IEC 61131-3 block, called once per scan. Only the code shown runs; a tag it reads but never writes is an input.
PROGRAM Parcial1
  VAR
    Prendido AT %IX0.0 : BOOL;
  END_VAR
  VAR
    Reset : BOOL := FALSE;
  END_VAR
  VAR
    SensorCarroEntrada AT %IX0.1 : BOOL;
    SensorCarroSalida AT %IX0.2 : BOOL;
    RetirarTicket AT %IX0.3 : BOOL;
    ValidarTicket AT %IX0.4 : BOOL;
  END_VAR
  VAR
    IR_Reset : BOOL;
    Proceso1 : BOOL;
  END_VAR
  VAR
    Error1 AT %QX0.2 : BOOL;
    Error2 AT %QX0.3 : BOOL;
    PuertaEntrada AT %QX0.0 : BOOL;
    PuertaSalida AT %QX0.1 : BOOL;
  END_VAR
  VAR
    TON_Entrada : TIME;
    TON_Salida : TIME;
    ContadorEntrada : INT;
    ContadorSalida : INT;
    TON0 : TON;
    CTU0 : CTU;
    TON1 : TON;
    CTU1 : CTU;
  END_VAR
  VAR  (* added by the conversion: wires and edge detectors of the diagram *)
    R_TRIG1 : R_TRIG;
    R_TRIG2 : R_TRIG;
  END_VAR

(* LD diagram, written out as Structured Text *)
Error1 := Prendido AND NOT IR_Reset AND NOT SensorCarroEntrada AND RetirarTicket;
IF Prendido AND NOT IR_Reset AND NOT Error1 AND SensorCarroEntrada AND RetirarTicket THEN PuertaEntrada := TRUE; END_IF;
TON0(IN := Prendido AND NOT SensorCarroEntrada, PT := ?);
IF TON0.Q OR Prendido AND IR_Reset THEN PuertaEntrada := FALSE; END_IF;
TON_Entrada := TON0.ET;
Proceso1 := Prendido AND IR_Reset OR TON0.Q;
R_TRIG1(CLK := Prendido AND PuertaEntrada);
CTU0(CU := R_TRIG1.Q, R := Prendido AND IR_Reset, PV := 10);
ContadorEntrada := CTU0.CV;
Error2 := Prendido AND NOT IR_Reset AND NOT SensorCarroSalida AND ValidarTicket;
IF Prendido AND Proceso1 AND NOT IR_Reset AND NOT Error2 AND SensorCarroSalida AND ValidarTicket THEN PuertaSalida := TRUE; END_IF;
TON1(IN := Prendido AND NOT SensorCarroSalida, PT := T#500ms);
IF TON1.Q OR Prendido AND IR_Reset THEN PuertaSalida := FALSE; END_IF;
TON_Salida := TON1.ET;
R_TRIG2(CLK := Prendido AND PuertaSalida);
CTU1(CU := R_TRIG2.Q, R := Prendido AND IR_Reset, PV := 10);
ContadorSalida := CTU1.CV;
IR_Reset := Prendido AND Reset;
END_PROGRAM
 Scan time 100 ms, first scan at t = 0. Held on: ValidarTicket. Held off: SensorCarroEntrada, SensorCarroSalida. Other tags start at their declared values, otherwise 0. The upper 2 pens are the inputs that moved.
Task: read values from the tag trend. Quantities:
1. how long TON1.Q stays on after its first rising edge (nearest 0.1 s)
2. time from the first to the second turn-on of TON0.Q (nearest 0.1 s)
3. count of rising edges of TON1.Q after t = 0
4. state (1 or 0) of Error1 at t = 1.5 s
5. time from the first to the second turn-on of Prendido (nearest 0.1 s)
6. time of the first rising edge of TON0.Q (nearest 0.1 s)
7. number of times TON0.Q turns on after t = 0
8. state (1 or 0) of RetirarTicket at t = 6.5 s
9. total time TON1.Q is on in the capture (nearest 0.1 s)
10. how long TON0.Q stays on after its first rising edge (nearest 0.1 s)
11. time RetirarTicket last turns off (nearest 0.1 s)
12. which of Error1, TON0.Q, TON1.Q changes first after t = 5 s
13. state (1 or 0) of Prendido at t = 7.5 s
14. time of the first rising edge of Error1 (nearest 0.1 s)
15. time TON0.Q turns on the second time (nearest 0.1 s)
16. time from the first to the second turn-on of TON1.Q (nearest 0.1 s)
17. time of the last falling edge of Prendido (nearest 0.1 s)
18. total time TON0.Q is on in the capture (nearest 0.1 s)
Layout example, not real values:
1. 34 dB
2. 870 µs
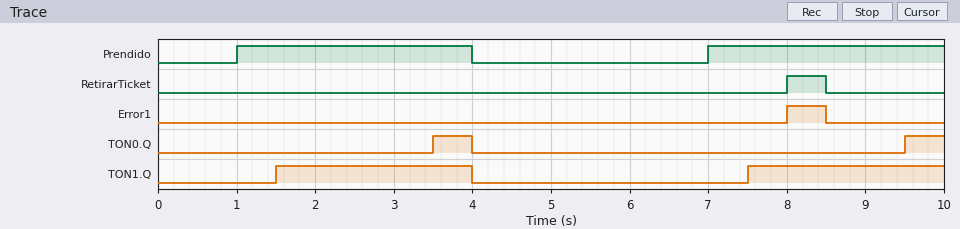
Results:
1. 2.5 s
2. 6.0 s
3. 2
4. 0
5. 6.0 s
6. 3.5 s
7. 2
8. 0
9. 5.0 s
10. 0.5 s
11. 8.5 s
12. TON1.Q
13. 1
14. 8.0 s
15. 9.5 s
16. 6.0 s
17. 4.0 s
18. 1.0 s
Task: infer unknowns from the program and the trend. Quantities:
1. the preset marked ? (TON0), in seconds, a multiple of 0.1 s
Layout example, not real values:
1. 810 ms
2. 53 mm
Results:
1. 2.5 s
